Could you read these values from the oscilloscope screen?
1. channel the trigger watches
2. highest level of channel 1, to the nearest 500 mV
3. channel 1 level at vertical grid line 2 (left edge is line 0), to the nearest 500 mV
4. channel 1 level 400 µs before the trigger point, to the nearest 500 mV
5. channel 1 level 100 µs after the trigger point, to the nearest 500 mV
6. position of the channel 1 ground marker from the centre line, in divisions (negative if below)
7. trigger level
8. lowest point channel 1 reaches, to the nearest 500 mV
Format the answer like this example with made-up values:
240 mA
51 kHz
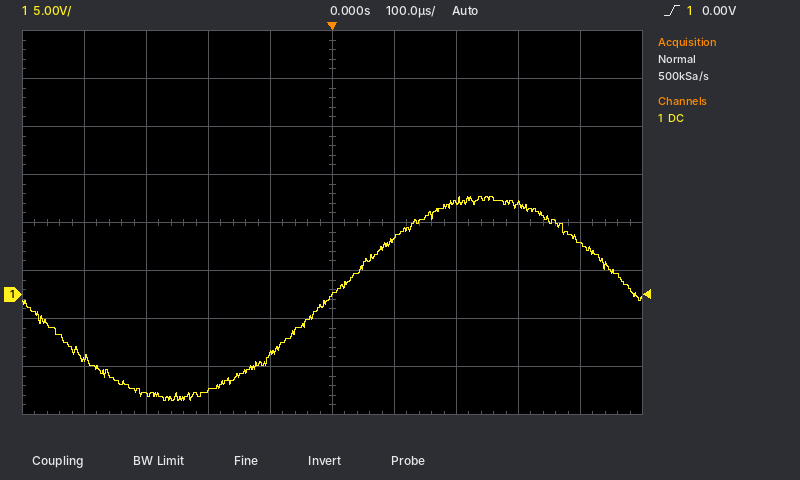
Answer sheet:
channel 1
10.0 V
-10.5 V
-6.5 V
6.0 V
-1.5 div
0.00 V
-11.0 V
